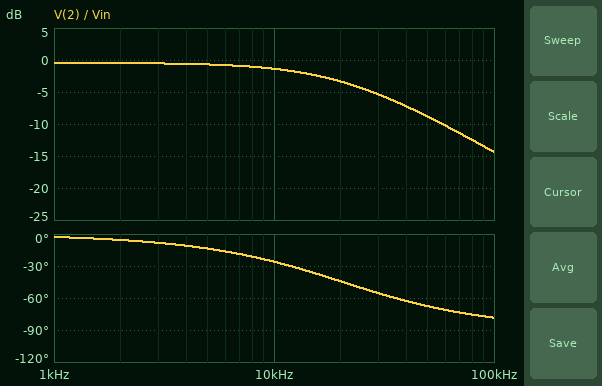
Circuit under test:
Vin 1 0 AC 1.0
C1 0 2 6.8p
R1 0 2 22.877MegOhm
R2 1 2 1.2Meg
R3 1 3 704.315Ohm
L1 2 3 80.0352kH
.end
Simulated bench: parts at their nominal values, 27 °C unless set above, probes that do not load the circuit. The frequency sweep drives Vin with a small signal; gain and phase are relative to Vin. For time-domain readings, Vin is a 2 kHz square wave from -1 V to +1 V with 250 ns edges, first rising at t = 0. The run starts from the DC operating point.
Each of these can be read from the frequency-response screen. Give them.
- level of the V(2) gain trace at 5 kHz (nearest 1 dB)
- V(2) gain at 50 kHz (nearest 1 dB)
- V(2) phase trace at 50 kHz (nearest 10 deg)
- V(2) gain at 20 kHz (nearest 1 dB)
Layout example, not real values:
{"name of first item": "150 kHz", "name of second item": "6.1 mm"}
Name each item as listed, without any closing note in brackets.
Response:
{"level of the V(2) gain trace at 5 kHz": "-1 dB", "V(2) gain at 50 kHz": "-9 dB", "V(2) phase trace at 50 kHz": "-70 deg", "V(2) gain at 20 kHz": "-3 dB"}
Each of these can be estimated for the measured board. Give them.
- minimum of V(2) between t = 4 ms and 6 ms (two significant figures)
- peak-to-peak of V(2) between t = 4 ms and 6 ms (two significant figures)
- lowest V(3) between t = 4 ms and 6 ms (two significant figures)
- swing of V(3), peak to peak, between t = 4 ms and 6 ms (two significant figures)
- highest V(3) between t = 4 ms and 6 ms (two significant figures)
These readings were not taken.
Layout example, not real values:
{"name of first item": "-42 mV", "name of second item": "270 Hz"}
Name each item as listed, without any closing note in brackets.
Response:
{"minimum of V(2) between t = 4 ms and 6 ms": "-1.0 V", "peak-to-peak of V(2) between t = 4 ms and 6 ms": "1.9 V", "lowest V(3) between t = 4 ms and 6 ms": "-1.0 V", "swing of V(3), peak to peak, between t = 4 ms and 6 ms": "2.0 V", "highest V(3) between t = 4 ms and 6 ms": "1.0 V"}
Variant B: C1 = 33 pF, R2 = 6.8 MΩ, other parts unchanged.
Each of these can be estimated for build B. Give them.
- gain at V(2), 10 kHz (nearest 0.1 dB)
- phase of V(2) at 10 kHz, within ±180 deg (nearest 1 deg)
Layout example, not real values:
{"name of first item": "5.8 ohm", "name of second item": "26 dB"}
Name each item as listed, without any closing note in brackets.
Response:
{"gain at V(2), 10 kHz": "-23.0 dB", "phase of V(2) at 10 kHz, within ±180 deg": "-85 deg"}
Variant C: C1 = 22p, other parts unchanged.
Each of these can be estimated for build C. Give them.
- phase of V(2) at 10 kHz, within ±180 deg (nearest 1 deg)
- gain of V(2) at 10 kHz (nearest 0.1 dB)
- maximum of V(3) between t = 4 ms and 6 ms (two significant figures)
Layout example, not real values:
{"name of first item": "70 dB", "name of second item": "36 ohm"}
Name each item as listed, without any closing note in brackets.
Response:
{"phase of V(2) at 10 kHz, within ±180 deg": "-58 deg", "gain of V(2) at 10 kHz": "-5.9 dB", "maximum of V(3) between t = 4 ms and 6 ms": "1.0 V"}
